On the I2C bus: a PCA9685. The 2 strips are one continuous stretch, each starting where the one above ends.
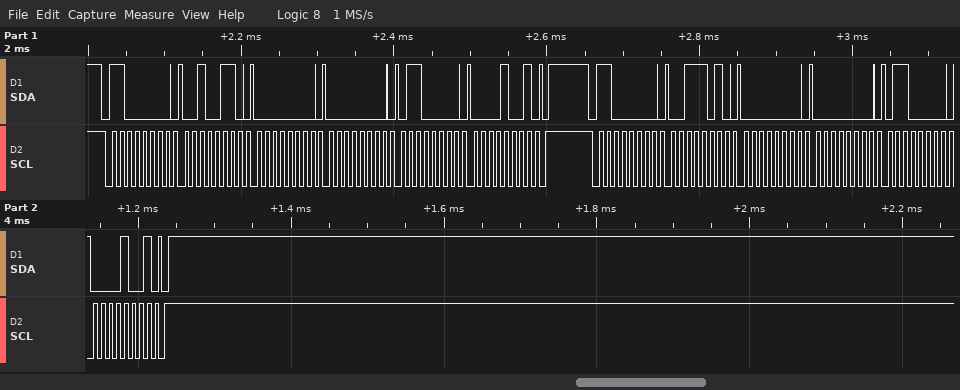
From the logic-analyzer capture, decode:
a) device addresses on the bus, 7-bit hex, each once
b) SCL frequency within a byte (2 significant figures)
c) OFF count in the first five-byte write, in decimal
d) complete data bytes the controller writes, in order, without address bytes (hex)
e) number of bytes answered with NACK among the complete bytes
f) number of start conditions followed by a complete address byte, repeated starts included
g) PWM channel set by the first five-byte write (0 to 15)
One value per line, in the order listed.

0x60
100 kHz
2400
26 00 00 60 09 3A 00 00 60 09
0
2
8
